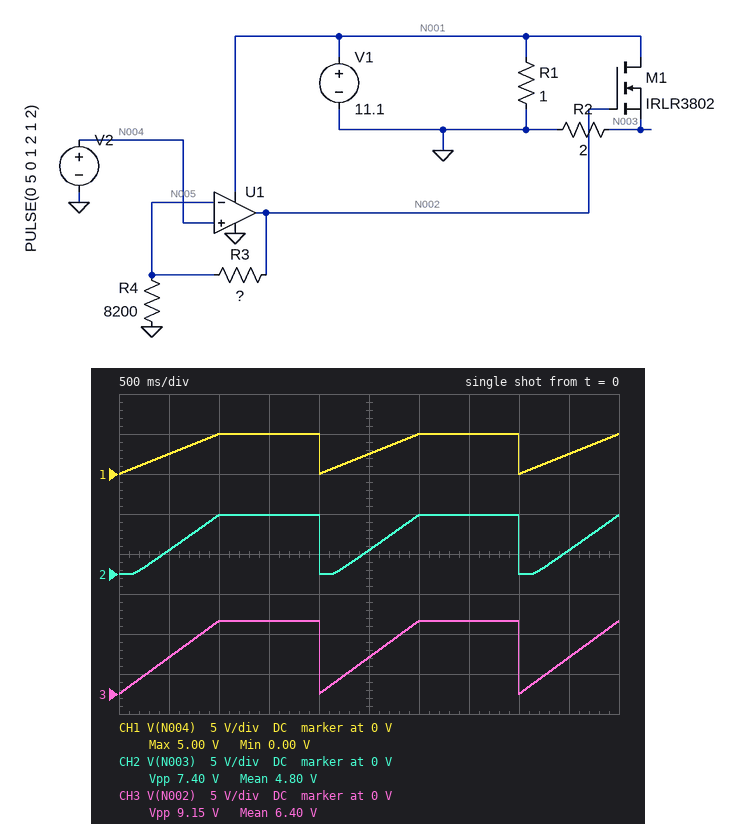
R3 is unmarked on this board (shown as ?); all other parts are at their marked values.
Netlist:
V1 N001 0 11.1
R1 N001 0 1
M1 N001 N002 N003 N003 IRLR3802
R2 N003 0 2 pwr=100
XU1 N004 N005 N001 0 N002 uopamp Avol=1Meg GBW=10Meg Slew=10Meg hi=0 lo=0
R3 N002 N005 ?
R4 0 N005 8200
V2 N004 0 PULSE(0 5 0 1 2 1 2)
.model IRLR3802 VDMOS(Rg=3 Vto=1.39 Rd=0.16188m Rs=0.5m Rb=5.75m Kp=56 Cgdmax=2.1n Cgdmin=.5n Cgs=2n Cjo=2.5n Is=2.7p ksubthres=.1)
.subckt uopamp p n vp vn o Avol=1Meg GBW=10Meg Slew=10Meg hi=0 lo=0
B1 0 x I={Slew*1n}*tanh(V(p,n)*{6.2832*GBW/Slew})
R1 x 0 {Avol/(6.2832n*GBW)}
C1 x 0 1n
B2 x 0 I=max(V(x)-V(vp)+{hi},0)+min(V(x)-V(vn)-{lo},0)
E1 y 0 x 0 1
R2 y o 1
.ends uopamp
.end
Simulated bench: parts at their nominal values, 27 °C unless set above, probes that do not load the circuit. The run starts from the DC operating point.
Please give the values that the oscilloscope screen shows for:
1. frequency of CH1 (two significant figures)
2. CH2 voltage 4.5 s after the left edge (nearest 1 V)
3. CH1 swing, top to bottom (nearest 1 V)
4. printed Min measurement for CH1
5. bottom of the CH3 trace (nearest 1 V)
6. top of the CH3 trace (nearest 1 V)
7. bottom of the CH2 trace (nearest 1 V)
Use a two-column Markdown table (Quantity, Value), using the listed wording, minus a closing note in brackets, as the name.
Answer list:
| Quantity | Value |
|---|---|
| frequency of CH1 | 500 mHz |
| CH2 voltage 4.5 s after the left edge | 3 V |
| CH1 swing, top to bottom | 5 V |
| printed Min measurement for CH1 | 0.00 V |
| bottom of the CH3 trace | 0 V |
| top of the CH3 trace | 9 V |
| bottom of the CH2 trace | 0 V |
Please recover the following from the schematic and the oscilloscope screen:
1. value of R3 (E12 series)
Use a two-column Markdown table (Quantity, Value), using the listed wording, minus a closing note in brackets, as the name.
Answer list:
| Quantity | Value |
|---|---|
| value of R3 | 6.8 kΩ |
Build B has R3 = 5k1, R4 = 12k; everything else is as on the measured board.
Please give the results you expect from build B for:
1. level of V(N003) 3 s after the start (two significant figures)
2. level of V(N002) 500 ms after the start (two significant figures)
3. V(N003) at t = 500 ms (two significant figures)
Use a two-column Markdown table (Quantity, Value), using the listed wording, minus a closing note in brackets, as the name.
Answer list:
| Quantity | Value |
|---|---|
| level of V(N003) 3 s after the start | 5.4 V |
| level of V(N002) 500 ms after the start | 3.6 V |
| V(N003) at t = 500 ms | 2.0 V |
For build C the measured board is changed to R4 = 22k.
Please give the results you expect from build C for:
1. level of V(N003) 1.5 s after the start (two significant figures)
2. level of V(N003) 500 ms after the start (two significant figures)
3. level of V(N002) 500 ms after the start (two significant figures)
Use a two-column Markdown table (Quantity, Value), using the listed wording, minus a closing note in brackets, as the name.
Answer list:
| Quantity | Value |
|---|---|
| level of V(N003) 1.5 s after the start | 4.9 V |
| level of V(N003) 500 ms after the start | 1.7 V |
| level of V(N002) 500 ms after the start | 3.3 V |
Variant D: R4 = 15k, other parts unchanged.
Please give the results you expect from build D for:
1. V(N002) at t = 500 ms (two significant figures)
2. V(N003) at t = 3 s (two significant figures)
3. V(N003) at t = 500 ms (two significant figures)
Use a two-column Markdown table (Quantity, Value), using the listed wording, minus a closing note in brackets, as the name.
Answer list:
| Quantity | Value |
|---|---|
| V(N002) at t = 500 ms | 3.6 V |
| V(N003) at t = 3 s | 5.6 V |
| V(N003) at t = 500 ms | 2.1 V |
